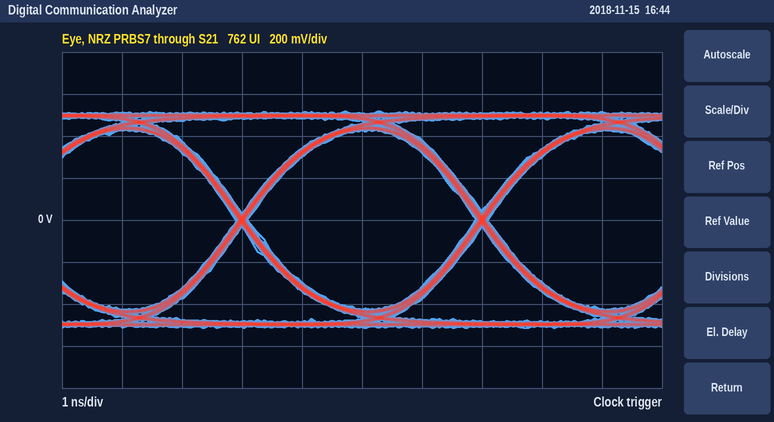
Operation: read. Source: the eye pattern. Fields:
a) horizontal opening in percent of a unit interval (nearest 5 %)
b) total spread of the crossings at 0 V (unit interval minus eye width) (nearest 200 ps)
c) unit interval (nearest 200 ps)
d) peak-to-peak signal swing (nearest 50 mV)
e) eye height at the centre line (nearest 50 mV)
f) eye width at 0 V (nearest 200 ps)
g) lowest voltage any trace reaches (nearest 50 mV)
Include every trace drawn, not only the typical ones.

95 %
200 ps
4.0 ns
1.05 V
850 mV
3.8 ns
-500 mV
